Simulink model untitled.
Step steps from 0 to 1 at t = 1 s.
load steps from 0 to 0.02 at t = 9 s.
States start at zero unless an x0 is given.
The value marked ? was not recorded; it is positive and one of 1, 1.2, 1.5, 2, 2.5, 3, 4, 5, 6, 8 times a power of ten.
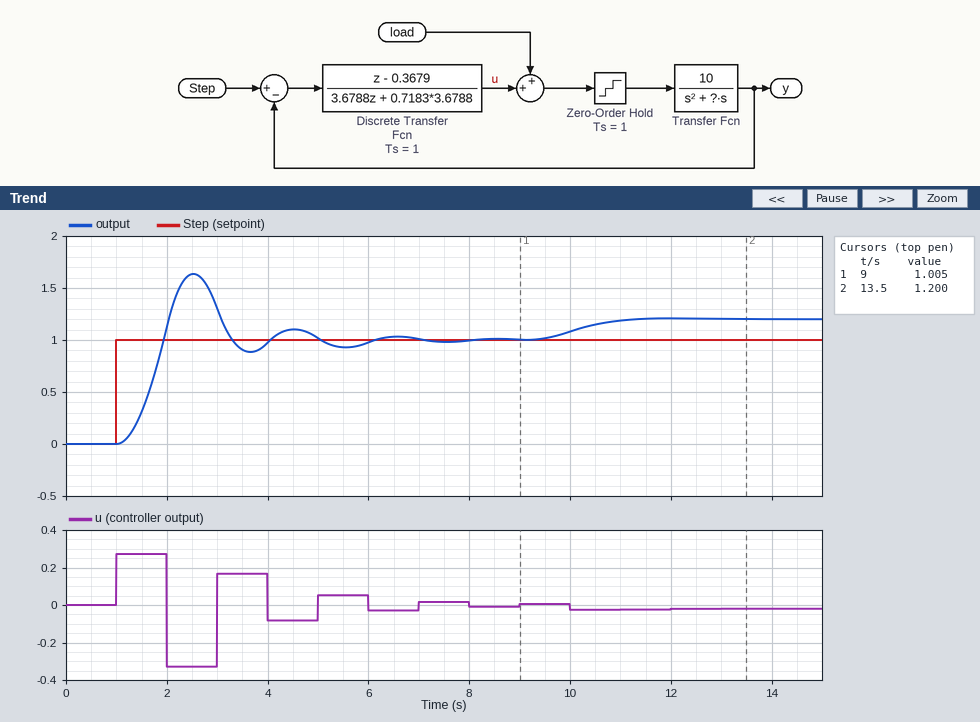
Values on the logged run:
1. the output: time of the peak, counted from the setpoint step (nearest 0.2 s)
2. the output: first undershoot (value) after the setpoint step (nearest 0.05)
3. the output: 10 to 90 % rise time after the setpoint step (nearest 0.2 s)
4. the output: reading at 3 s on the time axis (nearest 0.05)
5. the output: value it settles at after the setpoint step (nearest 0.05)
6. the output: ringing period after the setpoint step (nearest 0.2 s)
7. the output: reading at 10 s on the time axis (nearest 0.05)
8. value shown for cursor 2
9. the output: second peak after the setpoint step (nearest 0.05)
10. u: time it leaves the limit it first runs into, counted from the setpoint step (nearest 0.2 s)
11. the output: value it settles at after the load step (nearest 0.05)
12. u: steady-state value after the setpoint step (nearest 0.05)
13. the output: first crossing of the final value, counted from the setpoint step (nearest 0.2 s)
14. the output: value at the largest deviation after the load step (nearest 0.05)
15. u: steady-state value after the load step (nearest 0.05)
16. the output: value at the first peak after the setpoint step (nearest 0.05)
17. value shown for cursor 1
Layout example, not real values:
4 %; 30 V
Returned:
1.6 s; 0.90; 0.6 s; 1.30; 1.00; 2.0 s; 1.10; 1.200; 1.10; 1.0 s; 1.20; 0.00; 1.0 s; 1.20; 0.00; 1.65; 1.005
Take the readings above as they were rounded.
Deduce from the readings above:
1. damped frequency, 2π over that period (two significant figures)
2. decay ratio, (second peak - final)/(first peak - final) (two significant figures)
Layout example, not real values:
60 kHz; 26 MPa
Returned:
3.1 rad/s; 0.15
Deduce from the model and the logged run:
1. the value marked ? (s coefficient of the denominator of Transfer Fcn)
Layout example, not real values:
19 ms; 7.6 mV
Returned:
0.6
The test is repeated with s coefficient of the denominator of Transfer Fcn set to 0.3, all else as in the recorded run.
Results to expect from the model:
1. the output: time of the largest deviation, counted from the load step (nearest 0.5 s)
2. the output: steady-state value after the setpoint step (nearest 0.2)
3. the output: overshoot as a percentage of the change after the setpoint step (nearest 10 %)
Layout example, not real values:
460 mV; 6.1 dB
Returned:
2.5 s; 1.0; 90 %
